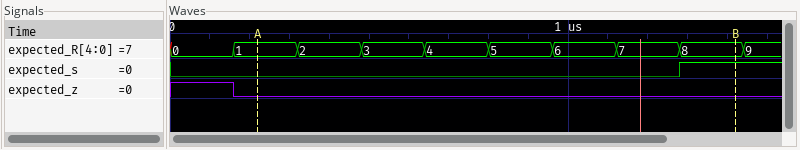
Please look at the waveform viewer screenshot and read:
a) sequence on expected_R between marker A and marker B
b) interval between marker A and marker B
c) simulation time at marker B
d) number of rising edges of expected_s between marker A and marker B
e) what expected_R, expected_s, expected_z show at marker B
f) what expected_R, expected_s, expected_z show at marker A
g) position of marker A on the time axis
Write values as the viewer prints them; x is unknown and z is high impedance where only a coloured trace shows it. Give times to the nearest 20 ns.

1, 2, 3, 4, 5, 6, 7, 8
1200 ns
1420 ns
1
expected_R=8, expected_s=1, expected_z=0
expected_R=1, expected_s=0, expected_z=0
220 ns
